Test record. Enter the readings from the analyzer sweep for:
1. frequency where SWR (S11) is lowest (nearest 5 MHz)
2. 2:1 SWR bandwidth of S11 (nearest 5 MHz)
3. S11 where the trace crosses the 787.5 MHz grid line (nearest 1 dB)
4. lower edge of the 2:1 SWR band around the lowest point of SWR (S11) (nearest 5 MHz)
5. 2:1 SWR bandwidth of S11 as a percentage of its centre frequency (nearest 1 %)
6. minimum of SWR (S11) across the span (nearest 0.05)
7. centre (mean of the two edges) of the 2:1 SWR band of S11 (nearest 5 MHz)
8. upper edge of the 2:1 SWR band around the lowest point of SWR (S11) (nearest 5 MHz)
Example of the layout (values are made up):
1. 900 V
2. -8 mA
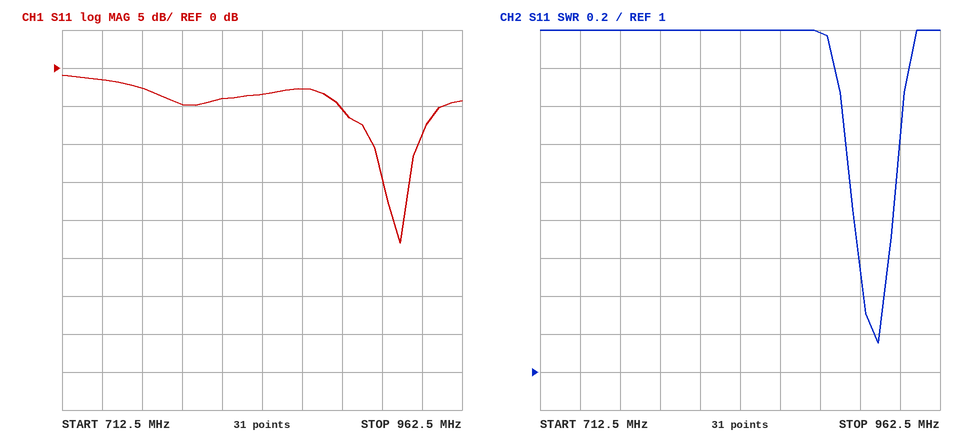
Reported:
1. 925 MHz
2. 30 MHz
3. -5 dB
4. 905 MHz
5. 3 %
6. 1.15
7. 920 MHz
8. 935 MHz
